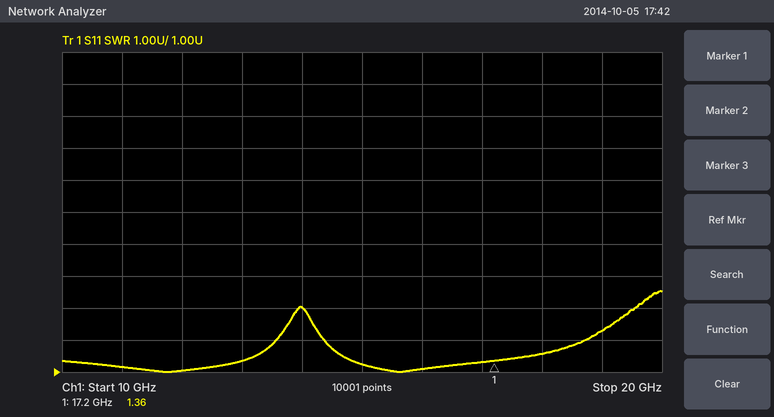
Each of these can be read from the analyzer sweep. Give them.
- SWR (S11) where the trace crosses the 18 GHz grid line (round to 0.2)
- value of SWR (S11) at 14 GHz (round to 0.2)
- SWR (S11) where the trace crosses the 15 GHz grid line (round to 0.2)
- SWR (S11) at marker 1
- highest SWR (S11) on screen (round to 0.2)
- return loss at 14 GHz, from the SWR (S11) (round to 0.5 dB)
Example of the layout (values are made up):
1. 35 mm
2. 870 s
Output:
1. 1.6
2. 3.0
3. 1.2
4. 1.36
5. 3.6
6. 6.0 dB
